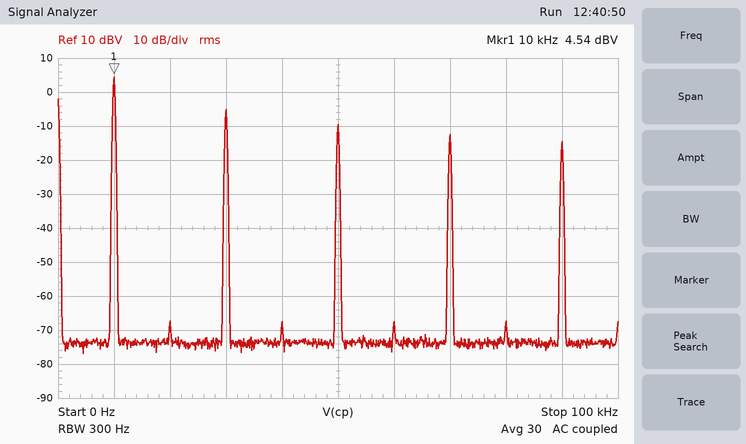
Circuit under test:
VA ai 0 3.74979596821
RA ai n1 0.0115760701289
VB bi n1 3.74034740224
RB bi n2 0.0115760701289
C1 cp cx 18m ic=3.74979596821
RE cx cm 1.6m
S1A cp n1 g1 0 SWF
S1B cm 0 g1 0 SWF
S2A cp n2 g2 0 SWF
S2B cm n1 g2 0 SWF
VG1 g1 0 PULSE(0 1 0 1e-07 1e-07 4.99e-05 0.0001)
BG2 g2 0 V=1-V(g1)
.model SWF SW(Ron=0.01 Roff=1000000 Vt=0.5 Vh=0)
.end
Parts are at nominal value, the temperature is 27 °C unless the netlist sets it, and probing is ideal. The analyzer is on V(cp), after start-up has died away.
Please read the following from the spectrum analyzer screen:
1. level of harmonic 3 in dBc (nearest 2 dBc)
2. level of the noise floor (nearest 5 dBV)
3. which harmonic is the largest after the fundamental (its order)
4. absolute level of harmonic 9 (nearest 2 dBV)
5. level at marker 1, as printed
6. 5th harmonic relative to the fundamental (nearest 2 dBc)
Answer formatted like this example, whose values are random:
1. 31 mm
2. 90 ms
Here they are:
1. -10 dBc
2. -75 dBV
3. 3
4. -14 dBV
5. 4.54 dBV
6. -14 dBc
